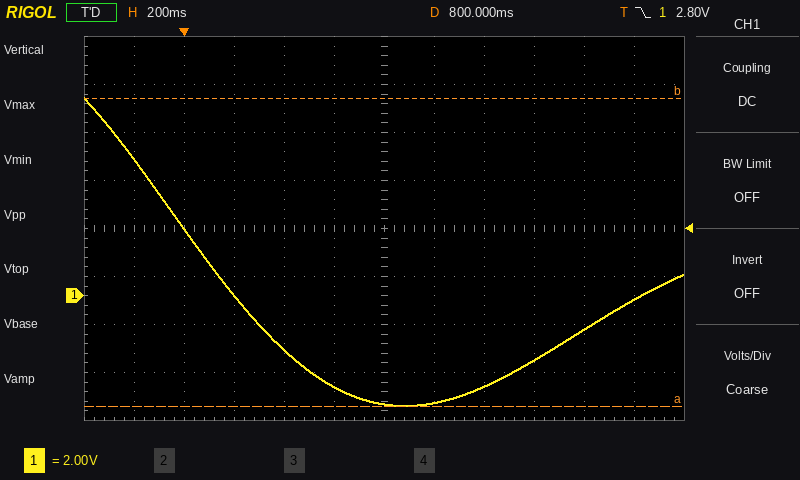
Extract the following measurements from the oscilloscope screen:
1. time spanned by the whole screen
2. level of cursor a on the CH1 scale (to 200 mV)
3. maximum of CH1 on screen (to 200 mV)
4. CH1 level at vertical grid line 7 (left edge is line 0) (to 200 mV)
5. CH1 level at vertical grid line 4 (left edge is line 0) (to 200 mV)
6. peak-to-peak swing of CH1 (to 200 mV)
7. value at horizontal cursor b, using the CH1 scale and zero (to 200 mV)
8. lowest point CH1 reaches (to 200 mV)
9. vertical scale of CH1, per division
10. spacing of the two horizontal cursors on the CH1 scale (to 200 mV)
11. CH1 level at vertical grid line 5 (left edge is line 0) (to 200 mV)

2.4 s
-4.6 V
8.2 V
-4.4 V
-2.2 V
12.8 V
8.2 V
-4.6 V
2 V
12.8 V
-3.8 V
